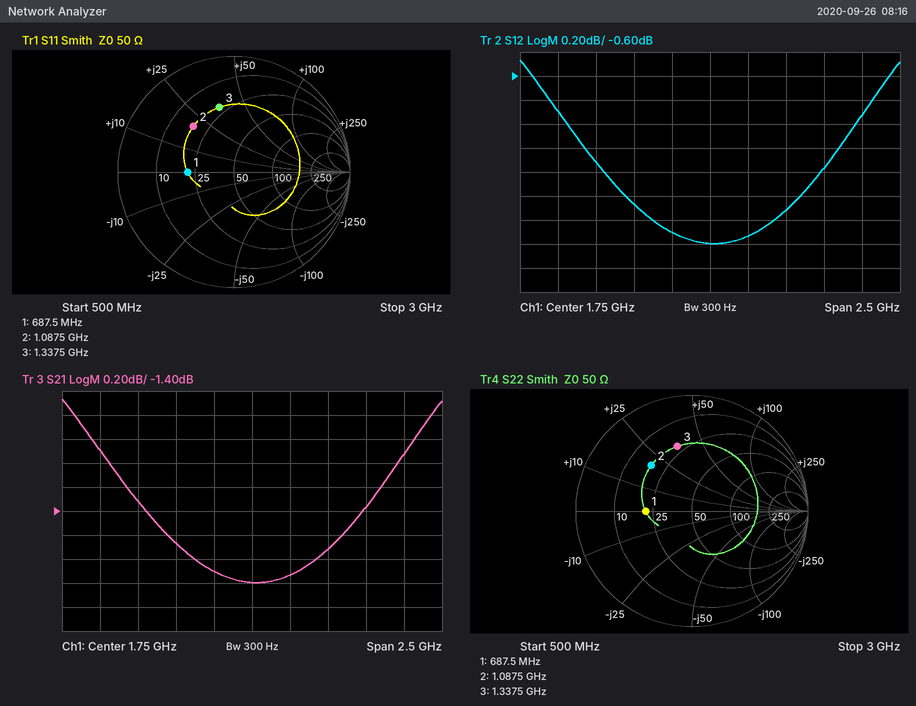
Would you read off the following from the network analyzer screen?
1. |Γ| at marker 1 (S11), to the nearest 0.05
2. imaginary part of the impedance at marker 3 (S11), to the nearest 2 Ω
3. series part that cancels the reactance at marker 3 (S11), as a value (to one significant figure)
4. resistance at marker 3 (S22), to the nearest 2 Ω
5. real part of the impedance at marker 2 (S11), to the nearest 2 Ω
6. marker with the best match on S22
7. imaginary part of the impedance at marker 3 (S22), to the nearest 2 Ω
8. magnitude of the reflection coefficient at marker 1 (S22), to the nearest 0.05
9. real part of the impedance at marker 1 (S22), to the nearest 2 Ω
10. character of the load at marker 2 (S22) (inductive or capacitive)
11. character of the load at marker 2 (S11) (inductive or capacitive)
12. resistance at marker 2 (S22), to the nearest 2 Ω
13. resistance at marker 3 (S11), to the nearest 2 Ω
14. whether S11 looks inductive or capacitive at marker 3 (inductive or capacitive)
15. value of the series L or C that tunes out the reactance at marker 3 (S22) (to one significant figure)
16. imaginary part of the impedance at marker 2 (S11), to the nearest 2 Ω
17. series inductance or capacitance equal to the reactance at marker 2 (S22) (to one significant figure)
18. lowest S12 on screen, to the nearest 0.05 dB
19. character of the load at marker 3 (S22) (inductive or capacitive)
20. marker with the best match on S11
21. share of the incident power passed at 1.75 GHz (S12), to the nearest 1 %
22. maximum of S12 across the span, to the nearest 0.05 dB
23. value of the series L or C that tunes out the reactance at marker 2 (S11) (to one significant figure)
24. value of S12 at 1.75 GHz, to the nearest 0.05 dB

0.40
+36 Ω
3 pF
22 Ω
18 Ω
marker 1
+36 Ω
0.40
22 Ω
inductive
inductive
18 Ω
22 Ω
inductive
3 pF
+20 Ω
3 nH
-2.00 dB
inductive
marker 1
63 %
-0.45 dB
7 pF
-2.00 dB
